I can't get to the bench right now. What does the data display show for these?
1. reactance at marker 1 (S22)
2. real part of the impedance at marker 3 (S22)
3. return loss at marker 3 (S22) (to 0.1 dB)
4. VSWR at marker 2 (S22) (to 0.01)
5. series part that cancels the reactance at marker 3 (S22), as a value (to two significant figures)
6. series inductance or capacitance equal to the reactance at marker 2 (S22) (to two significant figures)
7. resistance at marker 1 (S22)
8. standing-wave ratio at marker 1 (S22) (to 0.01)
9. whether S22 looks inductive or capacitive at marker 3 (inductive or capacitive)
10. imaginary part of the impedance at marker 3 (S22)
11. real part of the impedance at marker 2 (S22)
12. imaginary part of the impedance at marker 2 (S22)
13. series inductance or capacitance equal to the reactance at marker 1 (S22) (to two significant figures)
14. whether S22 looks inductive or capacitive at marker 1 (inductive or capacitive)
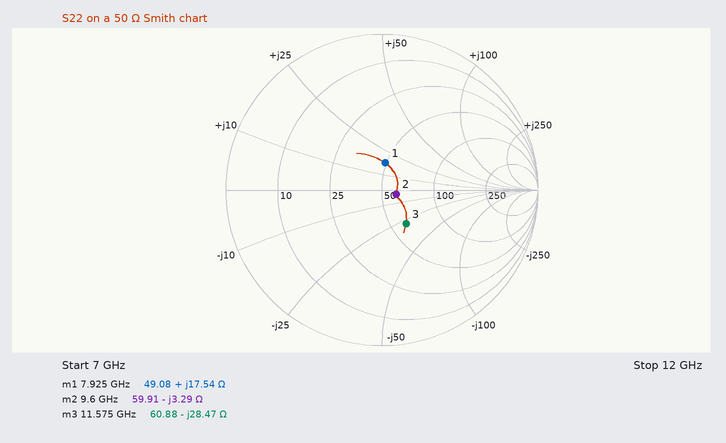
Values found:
+17.54 Ω
60.88 Ω
11.5 dB
1.21
390 pH
5.0 pF
49.08 Ω
1.42
capacitive
-28.47 Ω
59.91 Ω
-3.29 Ω
350 pH
inductive
